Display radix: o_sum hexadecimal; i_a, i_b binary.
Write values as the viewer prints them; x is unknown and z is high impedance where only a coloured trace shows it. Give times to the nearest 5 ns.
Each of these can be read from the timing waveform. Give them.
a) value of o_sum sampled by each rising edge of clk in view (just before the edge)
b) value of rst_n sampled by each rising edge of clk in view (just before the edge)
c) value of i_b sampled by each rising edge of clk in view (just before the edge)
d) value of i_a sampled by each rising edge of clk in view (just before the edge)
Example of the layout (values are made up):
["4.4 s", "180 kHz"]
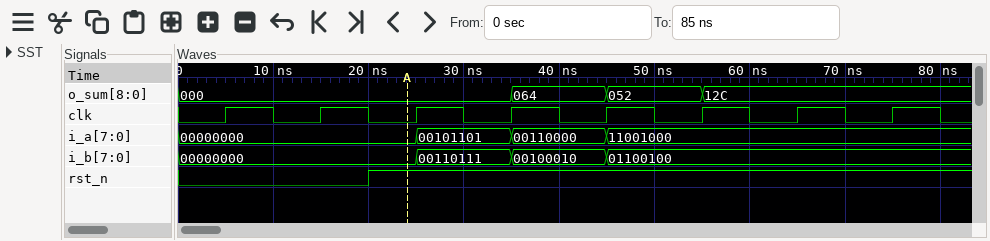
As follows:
["000, 000, 000, 000, 064, 052, 12C, 12C", "0 0 1 1 1 1 1 1", "00000000, 00000000, 00000000, 00110111, 00100010, 01100100, 01100100, 01100100", "00000000, 00000000, 00000000, 00101101, 00110000, 11001000, 11001000, 11001000"]
